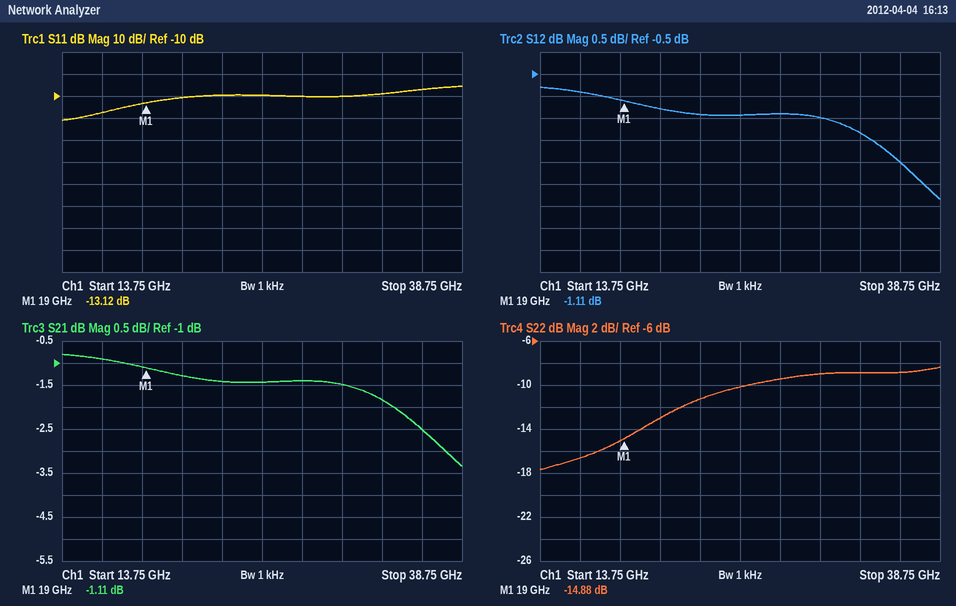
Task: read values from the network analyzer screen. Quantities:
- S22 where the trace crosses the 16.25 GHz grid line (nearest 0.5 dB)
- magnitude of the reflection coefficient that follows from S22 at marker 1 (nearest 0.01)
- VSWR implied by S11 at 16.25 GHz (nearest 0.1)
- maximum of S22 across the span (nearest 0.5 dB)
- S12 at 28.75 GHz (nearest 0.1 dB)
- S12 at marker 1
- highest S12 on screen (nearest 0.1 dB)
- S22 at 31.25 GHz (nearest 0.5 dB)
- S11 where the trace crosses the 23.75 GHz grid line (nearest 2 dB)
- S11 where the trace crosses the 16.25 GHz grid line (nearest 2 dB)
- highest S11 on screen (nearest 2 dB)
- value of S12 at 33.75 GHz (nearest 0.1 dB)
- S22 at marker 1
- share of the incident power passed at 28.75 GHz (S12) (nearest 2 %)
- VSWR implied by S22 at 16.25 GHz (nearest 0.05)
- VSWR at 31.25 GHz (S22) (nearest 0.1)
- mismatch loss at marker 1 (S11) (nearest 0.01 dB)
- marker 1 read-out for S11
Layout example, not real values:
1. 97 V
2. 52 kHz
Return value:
1. -16.5 dB
2. 0.18
3. 1.3
4. -8.5 dB
5. -1.4 dB
6. -1.11 dB
7. -0.8 dB
8. -9.0 dB
9. -10 dB
10. -18 dB
11. -6 dB
12. -1.8 dB
13. -14.88 dB
14. 72 %
15. 1.35
16. 2.1
17. 0.22 dB
18. -13.12 dB
